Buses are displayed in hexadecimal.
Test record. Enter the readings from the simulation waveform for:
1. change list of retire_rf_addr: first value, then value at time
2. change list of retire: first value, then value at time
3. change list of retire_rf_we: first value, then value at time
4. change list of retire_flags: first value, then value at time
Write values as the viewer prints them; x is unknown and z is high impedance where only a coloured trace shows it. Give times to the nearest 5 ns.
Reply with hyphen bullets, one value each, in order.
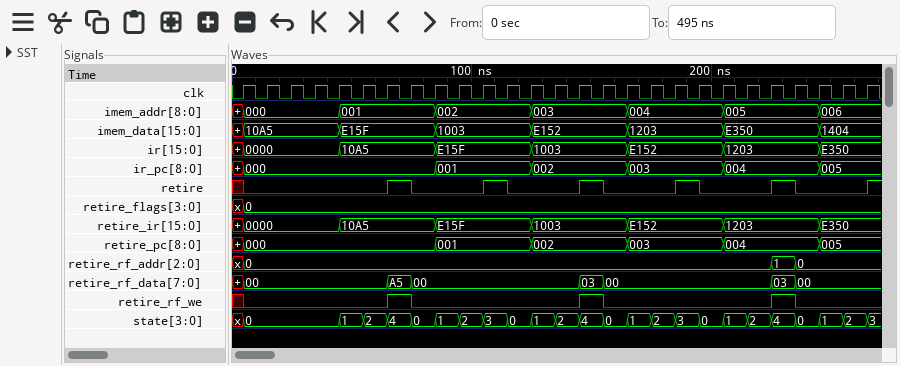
- x, 0 at 5 ns, 1 at 225 ns, 0 at 235 ns
- x, 0 at 5 ns, 1 at 65 ns, 0 at 75 ns, 1 at 105 ns, 0 at 115 ns, 1 at 145 ns, 0 at 155 ns, 1 at 185 ns, 0 at 195 ns, 1 at 225 ns, 0 at 235 ns, 1 at 265 ns
- x, 0 at 5 ns, 1 at 65 ns, 0 at 75 ns, 1 at 145 ns, 0 at 155 ns, 1 at 225 ns, 0 at 235 ns
- x, 0 at 5 ns
